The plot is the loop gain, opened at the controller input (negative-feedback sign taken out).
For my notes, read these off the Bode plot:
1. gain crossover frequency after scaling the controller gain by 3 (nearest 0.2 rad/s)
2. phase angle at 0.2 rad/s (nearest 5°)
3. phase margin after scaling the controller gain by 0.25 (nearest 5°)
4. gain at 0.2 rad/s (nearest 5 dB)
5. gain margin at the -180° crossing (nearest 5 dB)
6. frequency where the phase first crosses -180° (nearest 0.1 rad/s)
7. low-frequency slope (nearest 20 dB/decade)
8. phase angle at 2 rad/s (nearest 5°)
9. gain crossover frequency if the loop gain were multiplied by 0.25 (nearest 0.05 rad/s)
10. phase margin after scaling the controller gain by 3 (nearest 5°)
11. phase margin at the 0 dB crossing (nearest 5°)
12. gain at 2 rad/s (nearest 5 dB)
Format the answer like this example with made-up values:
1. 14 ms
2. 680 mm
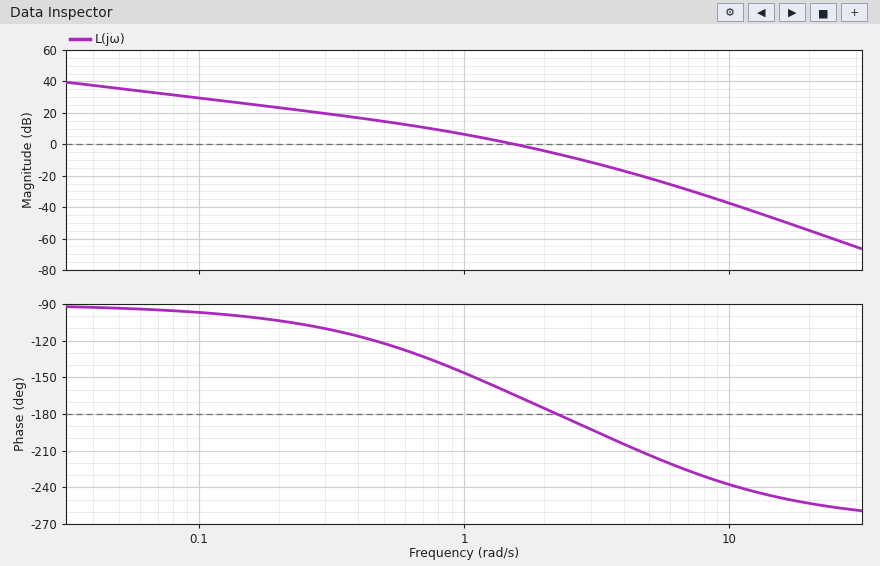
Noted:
1. 2.8 rad/s
2. -105°
3. 50°
4. 25 dB
5. 5 dB
6. 2.2 rad/s
7. -20 dB/decade
8. -175°
9. 0.65 rad/s
10. -10°
11. 15°
12. -5 dB
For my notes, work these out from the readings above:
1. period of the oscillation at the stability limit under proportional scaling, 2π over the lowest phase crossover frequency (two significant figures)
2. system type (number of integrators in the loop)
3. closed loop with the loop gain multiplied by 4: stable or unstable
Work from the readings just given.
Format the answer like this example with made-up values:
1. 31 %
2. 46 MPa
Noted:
1. 2.9 s
2. 1
3. unstable
